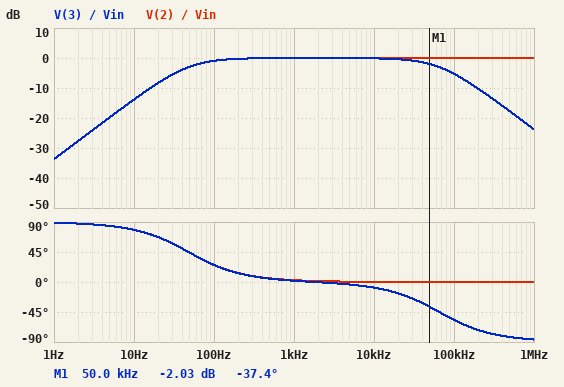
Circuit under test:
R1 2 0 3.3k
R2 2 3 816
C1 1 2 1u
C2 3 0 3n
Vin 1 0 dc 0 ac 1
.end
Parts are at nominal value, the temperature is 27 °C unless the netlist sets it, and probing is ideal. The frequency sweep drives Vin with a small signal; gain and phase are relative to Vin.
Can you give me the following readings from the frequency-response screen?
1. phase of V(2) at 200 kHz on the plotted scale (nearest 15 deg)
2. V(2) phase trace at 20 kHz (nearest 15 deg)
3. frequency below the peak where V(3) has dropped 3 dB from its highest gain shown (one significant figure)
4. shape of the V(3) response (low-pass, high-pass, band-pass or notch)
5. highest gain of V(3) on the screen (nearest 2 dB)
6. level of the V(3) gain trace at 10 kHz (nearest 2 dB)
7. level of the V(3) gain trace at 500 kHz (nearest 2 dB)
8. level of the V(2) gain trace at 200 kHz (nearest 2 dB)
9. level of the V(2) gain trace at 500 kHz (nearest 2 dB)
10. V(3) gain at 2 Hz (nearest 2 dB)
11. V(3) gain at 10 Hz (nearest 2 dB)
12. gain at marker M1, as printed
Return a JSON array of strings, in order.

["0 deg", "0 deg", "50 Hz", "band-pass", "0 dB", "0 dB", "-18 dB", "0 dB", "0 dB", "-28 dB", "-14 dB", "-2.03 dB"]
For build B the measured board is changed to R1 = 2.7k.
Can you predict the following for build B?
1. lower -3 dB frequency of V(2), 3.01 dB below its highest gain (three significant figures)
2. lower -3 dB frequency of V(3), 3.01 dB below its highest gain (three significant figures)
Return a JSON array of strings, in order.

["59.1 Hz", "58.7 Hz"]
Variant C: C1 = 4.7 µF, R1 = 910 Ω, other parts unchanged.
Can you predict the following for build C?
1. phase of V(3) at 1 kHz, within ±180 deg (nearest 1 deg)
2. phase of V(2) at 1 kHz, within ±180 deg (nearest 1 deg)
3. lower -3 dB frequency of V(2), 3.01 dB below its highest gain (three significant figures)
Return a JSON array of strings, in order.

["1 deg", "2 deg", "37.2 Hz"]
